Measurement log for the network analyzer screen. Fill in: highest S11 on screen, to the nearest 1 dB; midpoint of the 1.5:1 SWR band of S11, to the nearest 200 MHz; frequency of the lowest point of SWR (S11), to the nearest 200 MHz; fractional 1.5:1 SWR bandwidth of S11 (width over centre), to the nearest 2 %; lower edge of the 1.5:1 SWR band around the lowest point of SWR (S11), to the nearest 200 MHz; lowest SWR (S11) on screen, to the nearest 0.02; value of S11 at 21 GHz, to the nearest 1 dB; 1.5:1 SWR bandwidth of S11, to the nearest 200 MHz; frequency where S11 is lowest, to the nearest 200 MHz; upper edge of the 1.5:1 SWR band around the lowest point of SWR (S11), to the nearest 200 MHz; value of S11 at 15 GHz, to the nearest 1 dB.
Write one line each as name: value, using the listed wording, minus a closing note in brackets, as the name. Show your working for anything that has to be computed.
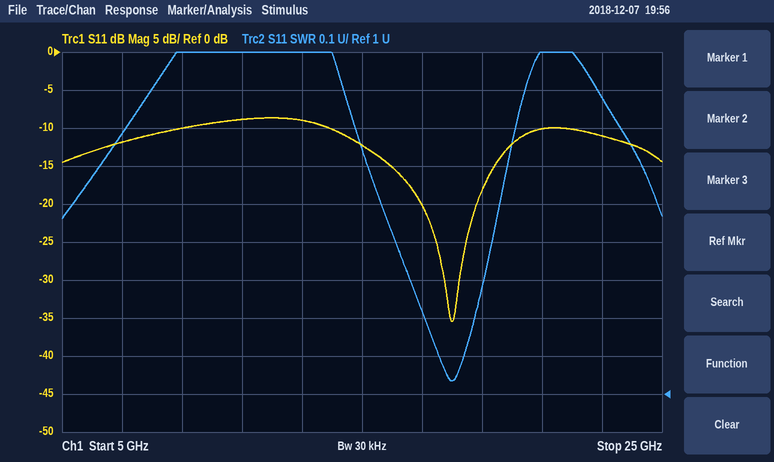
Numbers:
highest S11 on screen, to the nearest 1 dB: -9 dB
midpoint of the 1.5:1 SWR band of S11, to the nearest 200 MHz: 17.6 GHz
frequency of the lowest point of SWR (S11), to the nearest 200 MHz: 18.0 GHz
fractional 1.5:1 SWR bandwidth of S11 (width over centre), to the nearest 2 %: 4 GHz / 17.6 GHz ≈ 22.7 %, so 22 % to the nearest 2 %
lower edge of the 1.5:1 SWR band around the lowest point of SWR (S11), to the nearest 200 MHz: 15.6 GHz
lowest SWR (S11) on screen, to the nearest 0.02: 1.04
value of S11 at 21 GHz, to the nearest 1 dB: -10 dB
1.5:1 SWR bandwidth of S11, to the nearest 200 MHz: 19.6 GHz − 15.6 GHz = 4.0 GHz
frequency where S11 is lowest, to the nearest 200 MHz: 18.0 GHz
upper edge of the 1.5:1 SWR band around the lowest point of SWR (S11), to the nearest 200 MHz: 19.6 GHz
value of S11 at 15 GHz, to the nearest 1 dB: -12 dB
